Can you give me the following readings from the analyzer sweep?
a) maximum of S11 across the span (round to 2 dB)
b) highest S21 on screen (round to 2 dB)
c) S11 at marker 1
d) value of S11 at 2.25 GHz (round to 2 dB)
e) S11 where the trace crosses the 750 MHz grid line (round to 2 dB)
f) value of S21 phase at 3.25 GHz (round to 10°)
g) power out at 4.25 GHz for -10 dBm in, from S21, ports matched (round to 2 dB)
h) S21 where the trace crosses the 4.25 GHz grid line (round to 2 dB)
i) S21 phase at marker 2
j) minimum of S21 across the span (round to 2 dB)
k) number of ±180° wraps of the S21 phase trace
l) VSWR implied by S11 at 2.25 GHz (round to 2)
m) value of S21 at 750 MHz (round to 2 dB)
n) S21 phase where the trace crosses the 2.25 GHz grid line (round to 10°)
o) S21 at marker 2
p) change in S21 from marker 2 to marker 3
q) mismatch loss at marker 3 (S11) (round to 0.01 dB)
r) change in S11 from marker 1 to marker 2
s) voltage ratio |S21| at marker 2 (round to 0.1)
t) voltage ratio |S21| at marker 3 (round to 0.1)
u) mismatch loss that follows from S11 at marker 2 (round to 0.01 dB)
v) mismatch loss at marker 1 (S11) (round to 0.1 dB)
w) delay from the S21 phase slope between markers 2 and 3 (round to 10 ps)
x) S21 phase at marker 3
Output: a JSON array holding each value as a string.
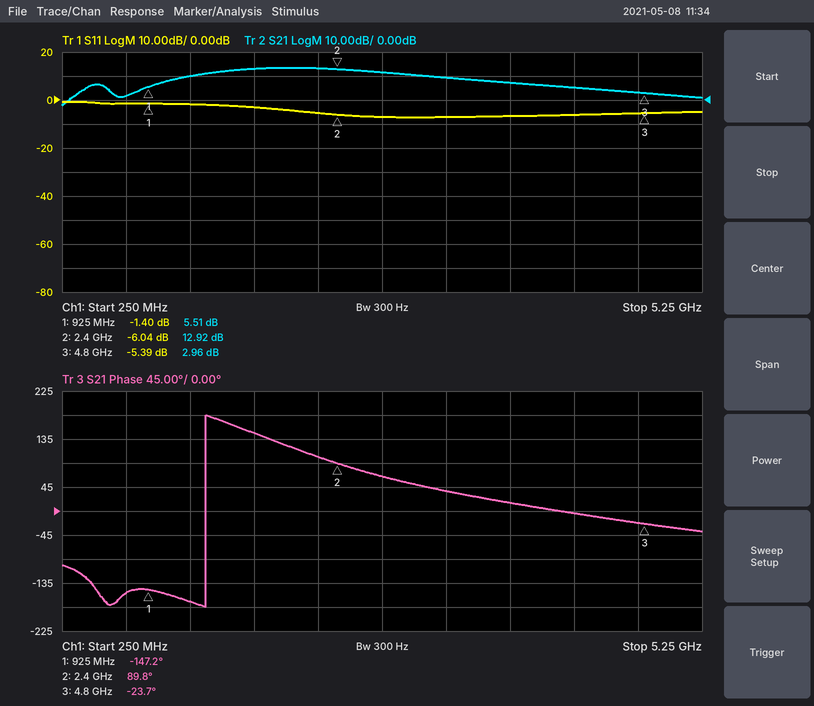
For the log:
["0 dB", "14 dB", "-1.40 dB", "-6 dB", "-2 dB", "40°", "-4 dBm", "6 dB", "89.8°", "-2 dB", "1", "4", "2 dB", "100°", "12.92 dB", "-9.96 dB", "1.48 dB", "-4.64 dB", "4.4", "1.4", "1.24 dB", "5.6 dB", "130 ps", "-23.7°"]
